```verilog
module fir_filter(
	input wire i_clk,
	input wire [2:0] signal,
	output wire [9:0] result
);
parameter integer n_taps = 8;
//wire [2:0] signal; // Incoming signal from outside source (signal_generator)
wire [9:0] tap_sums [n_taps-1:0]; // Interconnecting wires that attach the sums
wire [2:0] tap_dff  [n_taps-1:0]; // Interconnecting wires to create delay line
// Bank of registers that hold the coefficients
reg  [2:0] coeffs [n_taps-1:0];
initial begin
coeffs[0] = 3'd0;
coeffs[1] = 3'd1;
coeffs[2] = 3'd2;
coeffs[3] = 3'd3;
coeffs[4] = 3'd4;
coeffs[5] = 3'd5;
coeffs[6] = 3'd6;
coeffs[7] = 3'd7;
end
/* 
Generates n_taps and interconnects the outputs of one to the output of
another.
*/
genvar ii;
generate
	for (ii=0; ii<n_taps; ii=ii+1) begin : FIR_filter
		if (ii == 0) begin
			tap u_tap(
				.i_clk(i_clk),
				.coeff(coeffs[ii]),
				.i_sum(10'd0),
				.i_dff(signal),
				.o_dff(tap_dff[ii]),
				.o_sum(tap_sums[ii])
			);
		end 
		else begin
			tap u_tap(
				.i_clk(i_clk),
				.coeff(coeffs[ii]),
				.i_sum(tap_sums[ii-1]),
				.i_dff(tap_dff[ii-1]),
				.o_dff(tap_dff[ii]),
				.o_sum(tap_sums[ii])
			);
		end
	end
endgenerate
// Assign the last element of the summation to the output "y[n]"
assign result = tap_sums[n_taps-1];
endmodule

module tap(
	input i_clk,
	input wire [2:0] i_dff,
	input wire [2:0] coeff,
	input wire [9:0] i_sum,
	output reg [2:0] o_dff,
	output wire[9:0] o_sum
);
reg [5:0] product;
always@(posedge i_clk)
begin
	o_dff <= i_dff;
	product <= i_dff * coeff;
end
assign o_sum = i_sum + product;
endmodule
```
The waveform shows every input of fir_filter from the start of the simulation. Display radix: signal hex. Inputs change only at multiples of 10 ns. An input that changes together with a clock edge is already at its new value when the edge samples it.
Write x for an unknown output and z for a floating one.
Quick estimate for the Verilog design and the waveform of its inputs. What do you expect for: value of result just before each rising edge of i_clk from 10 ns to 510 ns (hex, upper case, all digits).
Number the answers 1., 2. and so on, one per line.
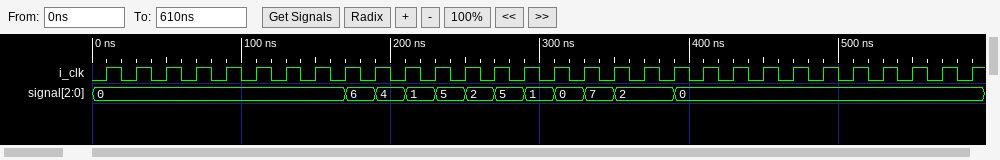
1. x, x, x, x, x, x, x, x, 000, 000, 006, 010, 01B, 02B, 03D, 054, 06C, 054, 04D, 05C, 04C, 04F, 038, 03C, 047, 01A
